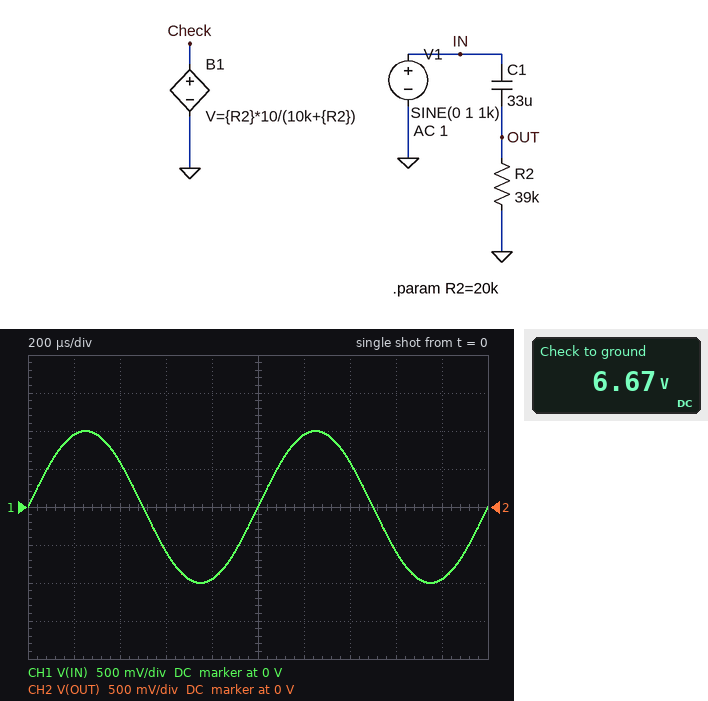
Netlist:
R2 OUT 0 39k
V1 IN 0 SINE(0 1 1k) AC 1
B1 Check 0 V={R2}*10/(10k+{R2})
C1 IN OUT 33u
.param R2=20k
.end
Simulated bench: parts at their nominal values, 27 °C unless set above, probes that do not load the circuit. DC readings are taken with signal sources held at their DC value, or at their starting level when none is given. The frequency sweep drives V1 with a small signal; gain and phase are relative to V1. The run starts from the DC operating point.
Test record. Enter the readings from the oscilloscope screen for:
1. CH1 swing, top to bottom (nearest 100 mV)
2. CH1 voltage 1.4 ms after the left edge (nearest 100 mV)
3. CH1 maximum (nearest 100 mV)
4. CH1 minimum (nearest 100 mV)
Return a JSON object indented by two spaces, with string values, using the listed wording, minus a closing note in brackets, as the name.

{
  "CH1 swing, top to bottom": "2.0 V",
  "CH1 voltage 1.4 ms after the left edge": "600 mV",
  "CH1 maximum": "1.0 V",
  "CH1 minimum": "-1.0 V"
}
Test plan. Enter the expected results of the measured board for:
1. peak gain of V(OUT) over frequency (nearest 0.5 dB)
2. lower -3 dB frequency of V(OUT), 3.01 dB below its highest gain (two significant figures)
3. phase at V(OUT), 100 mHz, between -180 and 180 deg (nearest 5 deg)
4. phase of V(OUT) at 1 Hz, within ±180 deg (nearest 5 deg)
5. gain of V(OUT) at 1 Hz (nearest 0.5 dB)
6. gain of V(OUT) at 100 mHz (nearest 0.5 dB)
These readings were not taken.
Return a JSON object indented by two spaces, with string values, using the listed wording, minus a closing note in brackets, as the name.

{
  "peak gain of V(OUT) over frequency": "0 dB",
  "lower -3 dB frequency of V(OUT), 3.01 dB below its highest gain": "120 mHz",
  "phase at V(OUT), 100 mHz, between -180 and 180 deg": "50 deg",
  "phase of V(OUT) at 1 Hz, within ±180 deg": "5 deg",
  "gain of V(OUT) at 1 Hz": "0 dB",
  "gain of V(OUT) at 100 mHz": "-4.0 dB"
}
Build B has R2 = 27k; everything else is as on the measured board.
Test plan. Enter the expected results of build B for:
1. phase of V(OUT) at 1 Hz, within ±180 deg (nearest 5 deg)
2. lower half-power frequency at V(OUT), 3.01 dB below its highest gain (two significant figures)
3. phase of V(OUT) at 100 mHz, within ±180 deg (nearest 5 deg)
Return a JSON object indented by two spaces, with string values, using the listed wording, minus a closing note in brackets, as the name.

{
  "phase of V(OUT) at 1 Hz, within ±180 deg": "10 deg",
  "lower half-power frequency at V(OUT), 3.01 dB below its highest gain": "180 mHz",
  "phase of V(OUT) at 100 mHz, within ±180 deg": "60 deg"
}
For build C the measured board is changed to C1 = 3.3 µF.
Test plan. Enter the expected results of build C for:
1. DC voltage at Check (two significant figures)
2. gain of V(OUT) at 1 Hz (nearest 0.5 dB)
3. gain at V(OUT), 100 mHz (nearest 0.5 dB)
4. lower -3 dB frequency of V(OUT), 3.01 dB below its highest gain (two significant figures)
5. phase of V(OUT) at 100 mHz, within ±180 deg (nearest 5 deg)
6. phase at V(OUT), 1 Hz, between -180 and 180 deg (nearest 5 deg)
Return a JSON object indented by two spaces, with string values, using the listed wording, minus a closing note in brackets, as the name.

{
  "DC voltage at Check": "6.7 V",
  "gain of V(OUT) at 1 Hz": "-4.0 dB",
  "gain at V(OUT), 100 mHz": "-22.0 dB",
  "lower -3 dB frequency of V(OUT), 3.01 dB below its highest gain": "1.2 Hz",
  "phase of V(OUT) at 100 mHz, within ±180 deg": "85 deg",
  "phase at V(OUT), 1 Hz, between -180 and 180 deg": "50 deg"
}
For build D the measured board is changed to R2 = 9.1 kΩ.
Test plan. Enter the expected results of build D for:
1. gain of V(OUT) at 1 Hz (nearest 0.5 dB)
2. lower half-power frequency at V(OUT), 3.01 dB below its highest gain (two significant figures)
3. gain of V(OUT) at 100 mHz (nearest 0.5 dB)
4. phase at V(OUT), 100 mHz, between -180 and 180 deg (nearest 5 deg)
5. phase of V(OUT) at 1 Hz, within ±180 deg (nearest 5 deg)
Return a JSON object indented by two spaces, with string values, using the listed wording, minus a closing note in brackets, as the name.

{
  "gain of V(OUT) at 1 Hz": "-1.0 dB",
  "lower half-power frequency at V(OUT), 3.01 dB below its highest gain": "530 mHz",
  "gain of V(OUT) at 100 mHz": "-14.5 dB",
  "phase at V(OUT), 100 mHz, between -180 and 180 deg": "80 deg",
  "phase of V(OUT) at 1 Hz, within ±180 deg": "30 deg"
}
